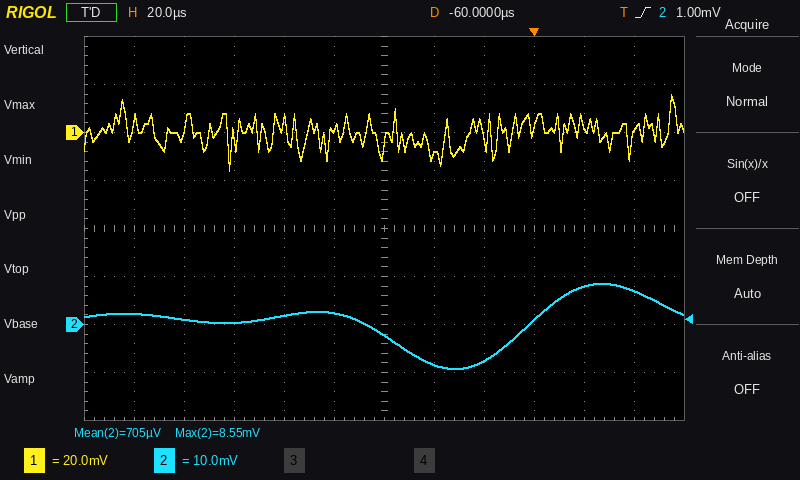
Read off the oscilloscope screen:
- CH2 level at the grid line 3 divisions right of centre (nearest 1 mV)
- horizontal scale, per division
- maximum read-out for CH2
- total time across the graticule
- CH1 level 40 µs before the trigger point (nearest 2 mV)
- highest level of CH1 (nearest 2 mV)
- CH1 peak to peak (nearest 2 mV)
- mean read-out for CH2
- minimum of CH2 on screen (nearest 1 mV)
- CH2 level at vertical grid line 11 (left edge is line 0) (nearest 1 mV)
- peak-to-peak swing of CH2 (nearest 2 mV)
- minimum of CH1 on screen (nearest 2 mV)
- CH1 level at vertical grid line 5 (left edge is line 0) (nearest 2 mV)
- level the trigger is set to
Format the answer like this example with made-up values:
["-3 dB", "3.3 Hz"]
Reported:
["1 mV", "20 µs", "8.55 mV", "240 µs", "-10 mV", "16 mV", "32 mV", "705 µV", "-9 mV", "7 mV", "18 mV", "-16 mV", "2 mV", "1.00 mV"]
